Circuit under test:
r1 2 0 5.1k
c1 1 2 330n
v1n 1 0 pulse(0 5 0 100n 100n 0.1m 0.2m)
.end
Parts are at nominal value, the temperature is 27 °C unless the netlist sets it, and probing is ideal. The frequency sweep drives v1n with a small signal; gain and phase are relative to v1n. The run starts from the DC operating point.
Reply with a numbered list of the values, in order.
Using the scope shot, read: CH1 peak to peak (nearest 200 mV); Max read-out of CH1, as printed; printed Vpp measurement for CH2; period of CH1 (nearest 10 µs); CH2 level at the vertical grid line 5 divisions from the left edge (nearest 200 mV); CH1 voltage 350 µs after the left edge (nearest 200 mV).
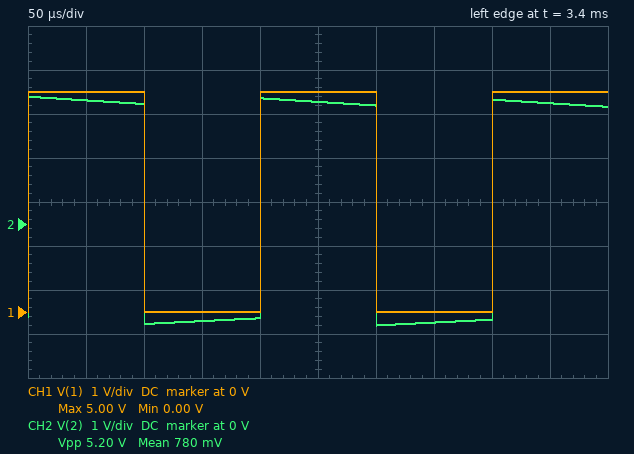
1. 5.0 V
2. 5.00 V
3. 5.20 V
4. 200 µs
5. 2.8 V
6. 0 V
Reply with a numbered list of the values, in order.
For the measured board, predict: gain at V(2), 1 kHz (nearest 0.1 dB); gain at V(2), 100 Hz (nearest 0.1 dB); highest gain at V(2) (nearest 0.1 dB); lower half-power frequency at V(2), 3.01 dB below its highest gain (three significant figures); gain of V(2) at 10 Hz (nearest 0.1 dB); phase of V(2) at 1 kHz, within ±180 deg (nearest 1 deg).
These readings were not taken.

1. 0 dB
2. -2.8 dB
3. 0 dB
4. 94.6 Hz
5. -19.6 dB
6. 5 deg
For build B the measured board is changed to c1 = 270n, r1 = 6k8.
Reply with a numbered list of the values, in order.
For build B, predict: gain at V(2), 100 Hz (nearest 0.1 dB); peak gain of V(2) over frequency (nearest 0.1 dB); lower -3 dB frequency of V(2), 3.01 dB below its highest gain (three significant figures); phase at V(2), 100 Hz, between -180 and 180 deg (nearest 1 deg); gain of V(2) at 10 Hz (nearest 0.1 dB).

1. -2.4 dB
2. 0 dB
3. 86.7 Hz
4. 41 deg
5. -18.8 dB
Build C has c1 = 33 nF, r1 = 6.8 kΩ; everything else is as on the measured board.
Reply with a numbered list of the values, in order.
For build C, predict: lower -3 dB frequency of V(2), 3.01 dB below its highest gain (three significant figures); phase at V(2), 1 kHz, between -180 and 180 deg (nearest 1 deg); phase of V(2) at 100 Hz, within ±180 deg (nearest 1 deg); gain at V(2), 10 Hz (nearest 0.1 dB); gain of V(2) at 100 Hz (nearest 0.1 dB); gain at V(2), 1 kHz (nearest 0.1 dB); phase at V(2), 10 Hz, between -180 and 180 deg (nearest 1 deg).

1. 709 Hz
2. 35 deg
3. 82 deg
4. -37.0 dB
5. -17.1 dB
6. -1.8 dB
7. 89 deg
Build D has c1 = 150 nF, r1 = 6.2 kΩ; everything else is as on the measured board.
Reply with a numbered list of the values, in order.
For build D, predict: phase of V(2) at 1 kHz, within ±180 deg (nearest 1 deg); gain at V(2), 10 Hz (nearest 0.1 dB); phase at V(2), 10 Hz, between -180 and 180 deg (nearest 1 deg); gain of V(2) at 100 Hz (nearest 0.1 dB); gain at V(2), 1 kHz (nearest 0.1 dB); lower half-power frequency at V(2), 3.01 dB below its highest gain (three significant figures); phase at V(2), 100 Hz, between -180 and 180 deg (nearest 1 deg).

1. 10 deg
2. -24.7 dB
3. 87 deg
4. -5.9 dB
5. -0.1 dB
6. 171 Hz
7. 60 deg
